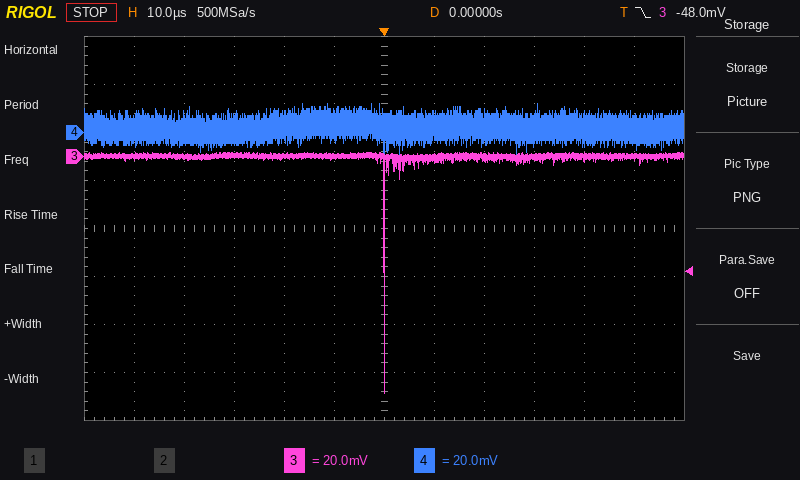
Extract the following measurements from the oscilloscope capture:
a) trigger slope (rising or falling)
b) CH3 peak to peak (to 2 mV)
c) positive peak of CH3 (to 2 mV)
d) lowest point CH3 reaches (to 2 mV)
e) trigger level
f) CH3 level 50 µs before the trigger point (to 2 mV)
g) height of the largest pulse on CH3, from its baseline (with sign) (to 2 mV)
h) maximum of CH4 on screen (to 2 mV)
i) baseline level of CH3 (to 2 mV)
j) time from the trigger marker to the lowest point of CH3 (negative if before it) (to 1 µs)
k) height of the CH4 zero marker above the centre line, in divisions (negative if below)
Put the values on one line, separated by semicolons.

falling; 100 mV; 2 mV; -98 mV; -48.0 mV; 0 mV; -98 mV; 12 mV; 0 mV; 0 µs; +2.0 div
